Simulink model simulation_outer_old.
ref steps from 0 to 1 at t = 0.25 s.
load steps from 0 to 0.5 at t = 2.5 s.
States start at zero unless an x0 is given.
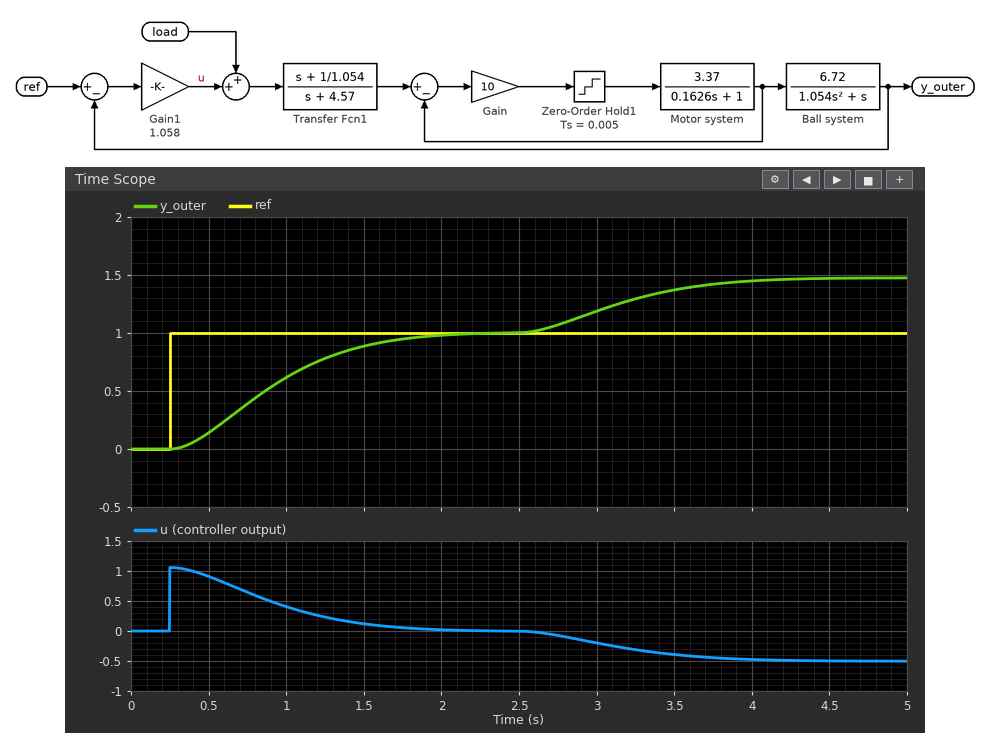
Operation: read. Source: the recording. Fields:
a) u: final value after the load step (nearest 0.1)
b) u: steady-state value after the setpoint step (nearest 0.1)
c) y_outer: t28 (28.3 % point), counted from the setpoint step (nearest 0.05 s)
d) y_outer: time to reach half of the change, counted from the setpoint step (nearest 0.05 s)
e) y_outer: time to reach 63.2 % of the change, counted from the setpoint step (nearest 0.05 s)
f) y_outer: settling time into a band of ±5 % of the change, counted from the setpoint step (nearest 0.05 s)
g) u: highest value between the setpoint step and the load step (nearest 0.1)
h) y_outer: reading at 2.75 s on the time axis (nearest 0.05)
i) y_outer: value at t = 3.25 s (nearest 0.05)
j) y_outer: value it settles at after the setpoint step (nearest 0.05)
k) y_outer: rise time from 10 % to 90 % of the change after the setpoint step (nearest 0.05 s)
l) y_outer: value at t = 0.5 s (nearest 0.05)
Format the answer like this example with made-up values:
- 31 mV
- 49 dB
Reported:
- -0.5
- 0.0
- 0.40 s
- 0.60 s
- 0.75 s
- 1.50 s
- 1.1
- 1.05
- 1.30
- 1.00
- 1.10 s
- 0.15
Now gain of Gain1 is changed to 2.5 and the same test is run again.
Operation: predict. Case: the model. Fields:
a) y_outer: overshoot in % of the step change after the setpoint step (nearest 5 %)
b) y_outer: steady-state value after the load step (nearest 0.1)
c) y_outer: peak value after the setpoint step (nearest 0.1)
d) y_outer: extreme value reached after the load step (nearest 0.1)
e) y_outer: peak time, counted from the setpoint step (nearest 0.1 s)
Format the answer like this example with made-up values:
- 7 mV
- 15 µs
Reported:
- 10 %
- 1.2
- 1.1
- 1.2
- 1.0 s
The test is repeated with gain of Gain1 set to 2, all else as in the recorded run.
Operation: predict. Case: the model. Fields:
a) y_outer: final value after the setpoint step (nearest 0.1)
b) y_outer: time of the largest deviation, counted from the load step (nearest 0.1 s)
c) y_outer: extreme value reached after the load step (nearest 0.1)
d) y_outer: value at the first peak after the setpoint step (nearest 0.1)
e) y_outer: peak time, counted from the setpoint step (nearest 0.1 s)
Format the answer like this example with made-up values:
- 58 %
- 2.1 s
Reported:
- 1.0
- 1.2 s
- 1.3
- 1.1
- 1.2 s
